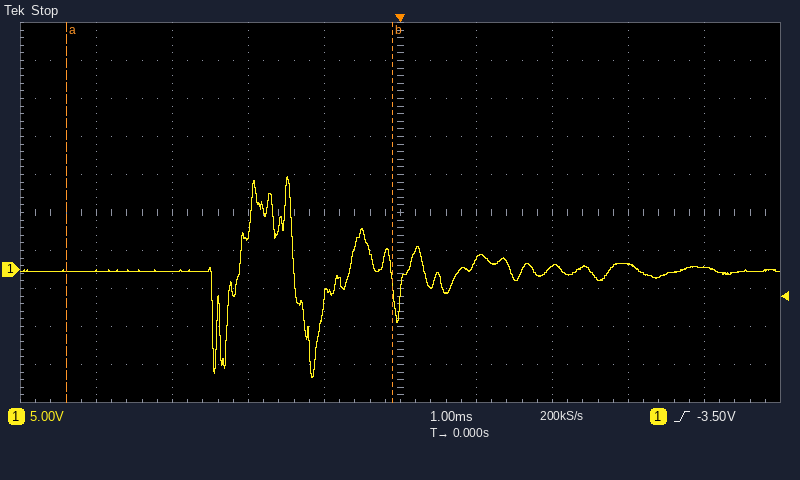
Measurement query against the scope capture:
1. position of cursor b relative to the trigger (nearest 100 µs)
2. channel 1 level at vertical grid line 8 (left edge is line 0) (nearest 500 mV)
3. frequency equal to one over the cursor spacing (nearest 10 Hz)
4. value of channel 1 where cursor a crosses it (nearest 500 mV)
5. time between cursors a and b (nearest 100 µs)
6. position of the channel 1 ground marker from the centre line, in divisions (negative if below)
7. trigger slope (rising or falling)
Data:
-100 µs
500 mV
230 Hz
0.0 V
4.3 ms
-1.5 div
rising
